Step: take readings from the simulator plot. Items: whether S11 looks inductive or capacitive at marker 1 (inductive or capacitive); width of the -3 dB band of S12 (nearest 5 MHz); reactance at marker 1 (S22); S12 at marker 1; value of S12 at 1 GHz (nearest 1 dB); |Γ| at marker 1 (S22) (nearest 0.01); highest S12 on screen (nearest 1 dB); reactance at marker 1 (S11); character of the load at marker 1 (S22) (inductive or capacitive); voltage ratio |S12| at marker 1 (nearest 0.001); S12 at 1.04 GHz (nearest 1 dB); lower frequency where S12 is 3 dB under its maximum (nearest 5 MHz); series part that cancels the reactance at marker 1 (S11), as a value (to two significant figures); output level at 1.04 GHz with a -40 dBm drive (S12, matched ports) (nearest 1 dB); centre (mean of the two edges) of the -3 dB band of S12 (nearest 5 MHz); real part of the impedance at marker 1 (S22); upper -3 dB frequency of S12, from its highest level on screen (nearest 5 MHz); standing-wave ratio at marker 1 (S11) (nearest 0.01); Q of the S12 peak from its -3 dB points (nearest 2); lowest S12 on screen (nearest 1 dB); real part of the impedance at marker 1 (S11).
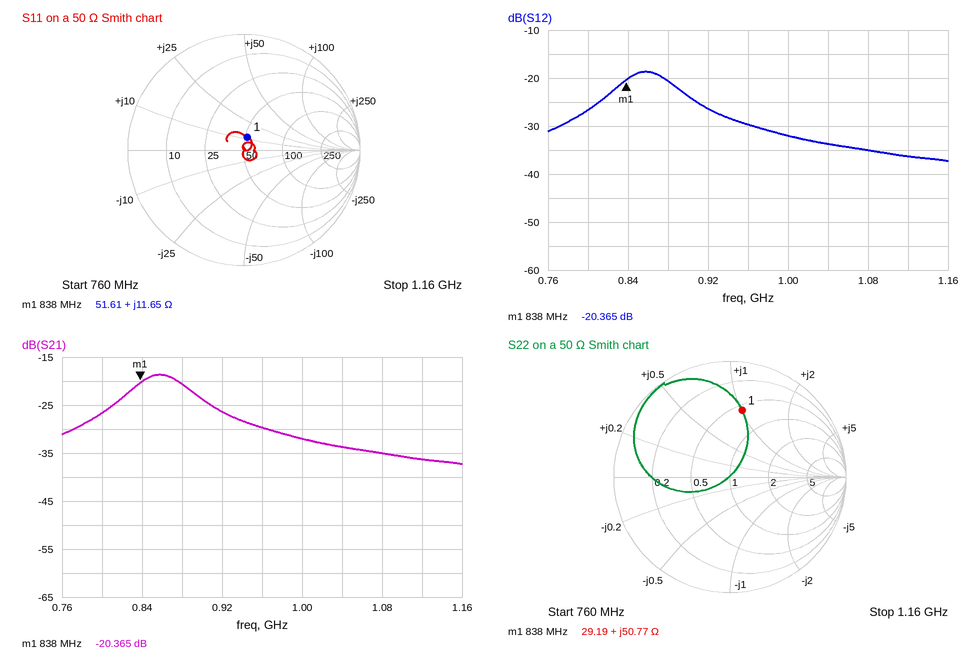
inductive
55 MHz
+50.77 Ω
-20.365 dB
-32 dB
0.58
-19 dB
+11.65 Ω
inductive
0.096
-34 dB
830 MHz
16 pF
-74 dBm
860 MHz
29.19 Ω
885 MHz
1.26
16
-37 dB
51.61 Ω
